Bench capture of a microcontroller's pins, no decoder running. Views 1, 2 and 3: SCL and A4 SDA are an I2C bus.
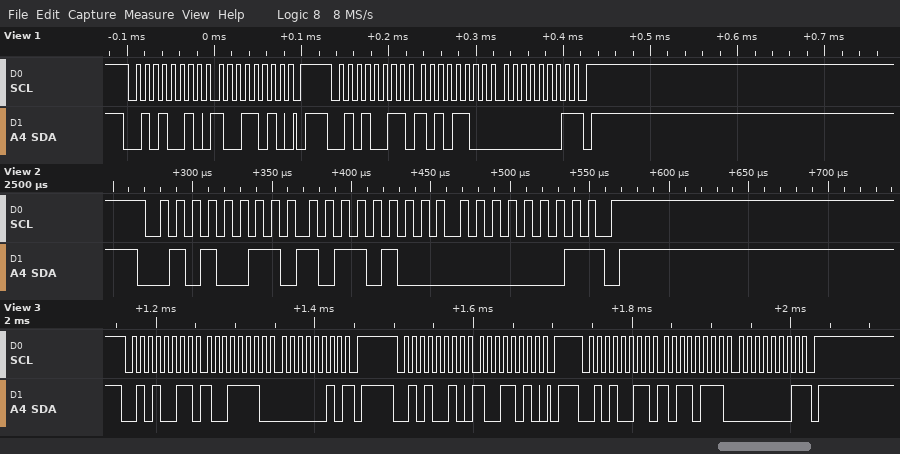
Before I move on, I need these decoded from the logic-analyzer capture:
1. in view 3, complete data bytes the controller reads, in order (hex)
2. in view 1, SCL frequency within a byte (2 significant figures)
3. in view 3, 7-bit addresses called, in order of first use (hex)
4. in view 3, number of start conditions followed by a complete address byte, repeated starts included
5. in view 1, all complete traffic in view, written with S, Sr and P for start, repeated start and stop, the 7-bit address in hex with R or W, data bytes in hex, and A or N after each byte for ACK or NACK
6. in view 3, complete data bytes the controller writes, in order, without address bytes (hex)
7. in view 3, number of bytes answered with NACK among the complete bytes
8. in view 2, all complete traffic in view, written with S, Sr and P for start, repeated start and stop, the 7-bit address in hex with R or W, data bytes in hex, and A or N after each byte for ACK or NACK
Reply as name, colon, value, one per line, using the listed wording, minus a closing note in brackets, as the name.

in view 3, complete data bytes the controller reads, in order: 9E 02 B7 01
in view 1, SCL frequency within a byte: 100 kHz
in view 3, 7-bit addresses called, in order of first use: 0x29
in view 3, number of start conditions followed by a complete address byte, repeated starts included: 3
in view 1, all complete traffic in view, written with S, Sr and P for start, repeated start and stop, the 7-bit address in hex with R or W, data bytes in hex, and A or N after each byte for ACK or NACK: S 29W A 9A A P S 29R A AC A 01 N P
in view 3, complete data bytes the controller writes, in order, without address bytes: 9A
in view 3, number of bytes answered with NACK among the complete bytes: 2
in view 2, all complete traffic in view, written with S, Sr and P for start, repeated start and stop, the 7-bit address in hex with R or W, data bytes in hex, and A or N after each byte for ACK or NACK: S 29R A B4 A 01 N P
